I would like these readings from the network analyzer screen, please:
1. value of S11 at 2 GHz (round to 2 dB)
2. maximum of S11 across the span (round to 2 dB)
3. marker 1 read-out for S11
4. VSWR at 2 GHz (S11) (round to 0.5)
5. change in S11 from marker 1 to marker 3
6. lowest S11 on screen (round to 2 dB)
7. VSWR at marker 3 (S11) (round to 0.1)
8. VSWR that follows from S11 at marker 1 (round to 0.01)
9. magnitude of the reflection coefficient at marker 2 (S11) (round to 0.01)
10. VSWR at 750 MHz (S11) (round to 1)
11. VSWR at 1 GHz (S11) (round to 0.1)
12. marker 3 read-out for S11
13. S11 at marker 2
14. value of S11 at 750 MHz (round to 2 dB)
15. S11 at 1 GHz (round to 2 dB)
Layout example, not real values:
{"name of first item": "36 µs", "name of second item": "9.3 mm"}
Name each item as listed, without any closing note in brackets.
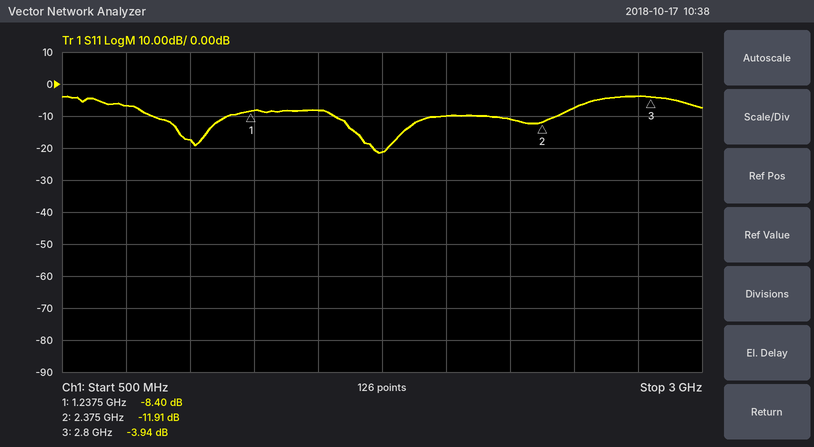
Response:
{"value of S11 at 2 GHz": "-10 dB", "maximum of S11 across the span": "-4 dB", "marker 1 read-out for S11": "-8.40 dB", "VSWR at 2 GHz (S11)": "2.0", "change in S11 from marker 1 to marker 3": "4.46 dB", "lowest S11 on screen": "-22 dB", "VSWR at marker 3 (S11)": "4.5", "VSWR that follows from S11 at marker 1": "2.23", "magnitude of the reflection coefficient at marker 2 (S11)": "0.25", "VSWR at 750 MHz (S11)": "3", "VSWR at 1 GHz (S11)": "1.3", "marker 3 read-out for S11": "-3.94 dB", "S11 at marker 2": "-11.91 dB", "value of S11 at 750 MHz": "-6 dB", "S11 at 1 GHz": "-18 dB"}
